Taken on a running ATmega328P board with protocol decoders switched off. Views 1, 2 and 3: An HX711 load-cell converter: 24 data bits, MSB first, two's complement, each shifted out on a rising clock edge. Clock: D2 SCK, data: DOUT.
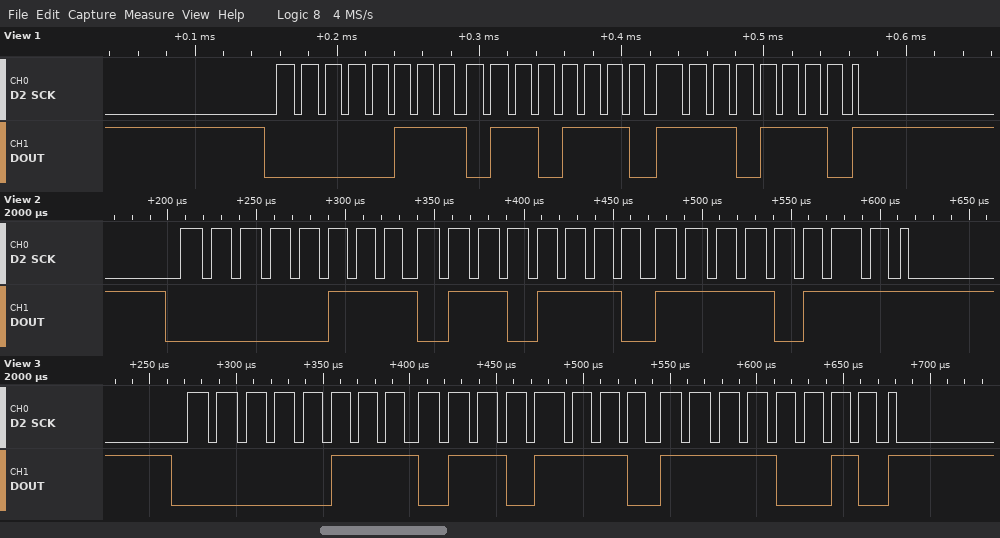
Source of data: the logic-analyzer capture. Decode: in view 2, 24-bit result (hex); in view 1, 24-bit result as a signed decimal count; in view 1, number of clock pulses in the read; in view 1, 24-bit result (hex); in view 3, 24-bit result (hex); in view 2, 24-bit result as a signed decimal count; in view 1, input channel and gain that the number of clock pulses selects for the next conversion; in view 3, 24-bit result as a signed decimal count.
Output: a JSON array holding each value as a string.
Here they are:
["0x076EF7", "487150", "25", "0x076EEE", "0x076EF2", "487159", "channel A, gain 128", "487154"]
